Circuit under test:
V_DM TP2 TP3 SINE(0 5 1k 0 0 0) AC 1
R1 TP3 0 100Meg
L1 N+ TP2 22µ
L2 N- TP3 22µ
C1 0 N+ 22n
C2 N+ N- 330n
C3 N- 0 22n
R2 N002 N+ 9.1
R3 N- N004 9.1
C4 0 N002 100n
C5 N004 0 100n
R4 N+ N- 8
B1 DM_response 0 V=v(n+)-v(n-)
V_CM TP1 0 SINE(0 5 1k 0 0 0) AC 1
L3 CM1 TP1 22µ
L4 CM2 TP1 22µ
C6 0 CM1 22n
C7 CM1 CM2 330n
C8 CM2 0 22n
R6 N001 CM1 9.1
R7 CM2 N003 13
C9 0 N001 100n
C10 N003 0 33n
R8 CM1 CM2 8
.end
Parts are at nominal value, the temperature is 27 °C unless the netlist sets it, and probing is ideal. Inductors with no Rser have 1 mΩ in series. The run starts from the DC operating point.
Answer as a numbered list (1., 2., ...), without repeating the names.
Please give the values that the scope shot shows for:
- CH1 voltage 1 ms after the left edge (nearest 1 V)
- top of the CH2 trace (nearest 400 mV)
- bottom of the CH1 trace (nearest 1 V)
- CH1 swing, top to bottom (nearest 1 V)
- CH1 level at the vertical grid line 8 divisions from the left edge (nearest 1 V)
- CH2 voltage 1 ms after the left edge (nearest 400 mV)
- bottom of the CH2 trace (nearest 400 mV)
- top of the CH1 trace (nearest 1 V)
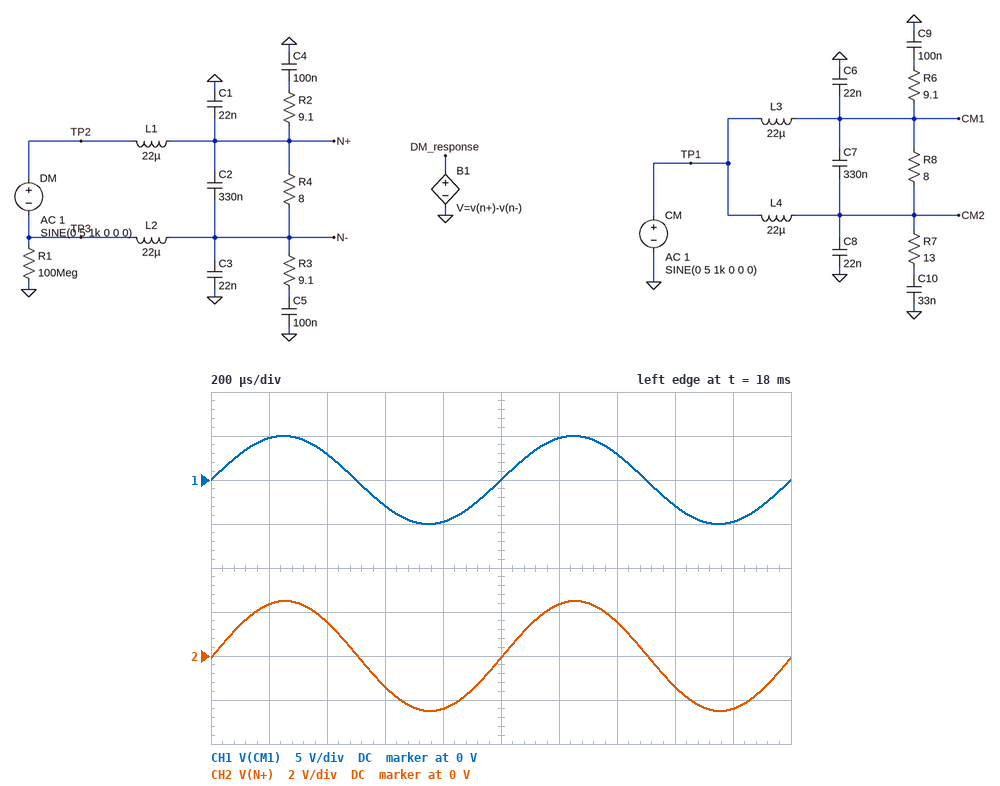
1. 0 V
2. 2.4 V
3. -5 V
4. 10 V
5. -3 V
6. 0 V
7. -2.4 V
8. 5 V
